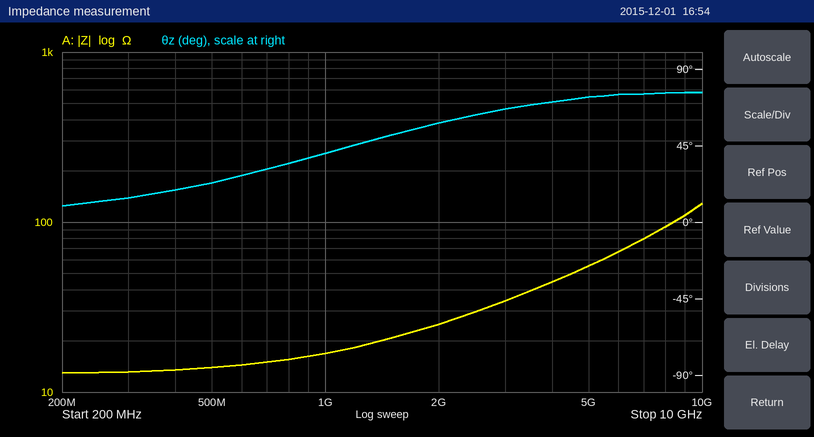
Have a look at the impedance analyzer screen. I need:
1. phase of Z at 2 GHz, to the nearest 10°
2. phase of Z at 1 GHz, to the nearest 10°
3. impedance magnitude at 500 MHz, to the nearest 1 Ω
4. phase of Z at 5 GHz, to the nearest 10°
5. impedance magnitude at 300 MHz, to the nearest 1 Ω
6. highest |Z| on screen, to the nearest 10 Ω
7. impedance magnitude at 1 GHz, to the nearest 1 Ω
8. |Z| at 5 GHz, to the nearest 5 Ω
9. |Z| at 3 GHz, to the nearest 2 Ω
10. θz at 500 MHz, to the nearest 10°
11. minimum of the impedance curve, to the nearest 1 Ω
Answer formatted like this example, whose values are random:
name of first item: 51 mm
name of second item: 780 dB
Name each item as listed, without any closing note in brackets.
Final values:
phase of Z at 2 GHz, to the nearest 10°: 60°
phase of Z at 1 GHz, to the nearest 10°: 40°
impedance magnitude at 500 MHz, to the nearest 1 Ω: 14 Ω
phase of Z at 5 GHz, to the nearest 10°: 70°
impedance magnitude at 300 MHz, to the nearest 1 Ω: 13 Ω
highest |Z| on screen, to the nearest 10 Ω: 130 Ω
impedance magnitude at 1 GHz, to the nearest 1 Ω: 17 Ω
|Z| at 5 GHz, to the nearest 5 Ω: 55 Ω
|Z| at 3 GHz, to the nearest 2 Ω: 34 Ω
θz at 500 MHz, to the nearest 10°: 20°
minimum of the impedance curve, to the nearest 1 Ω: 13 Ω
